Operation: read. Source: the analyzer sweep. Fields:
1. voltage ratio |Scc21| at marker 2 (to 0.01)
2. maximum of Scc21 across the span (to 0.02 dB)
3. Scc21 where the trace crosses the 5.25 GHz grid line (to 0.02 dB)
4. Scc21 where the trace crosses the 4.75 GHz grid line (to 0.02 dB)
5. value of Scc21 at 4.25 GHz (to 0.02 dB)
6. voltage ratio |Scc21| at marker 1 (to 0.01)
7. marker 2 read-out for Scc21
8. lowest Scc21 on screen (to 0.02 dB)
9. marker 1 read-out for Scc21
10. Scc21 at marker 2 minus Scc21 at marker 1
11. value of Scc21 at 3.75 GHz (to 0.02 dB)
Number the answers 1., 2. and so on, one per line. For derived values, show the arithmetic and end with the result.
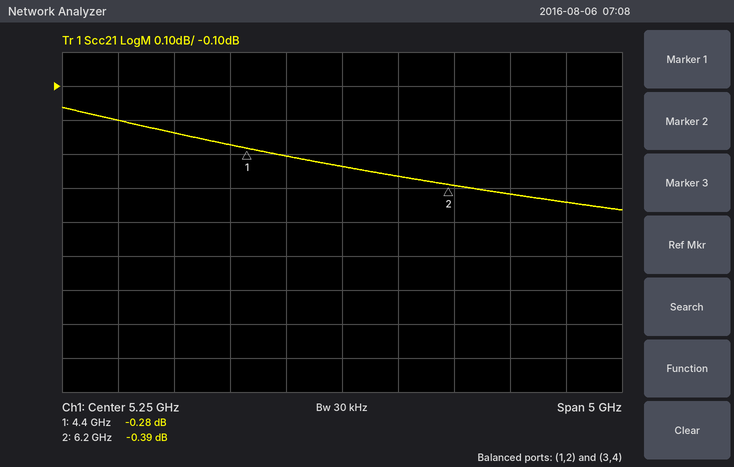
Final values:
1. 10^(-0.39/20) ≈ 0.96
2. -0.16 dB
3. -0.34 dB
4. -0.30 dB
5. -0.28 dB
6. 10^(-0.28/20) ≈ 0.97
7. -0.39 dB
8. -0.46 dB
9. -0.28 dB
10. -0.39 − (-0.28) = -0.11 dB
11. -0.24 dB
